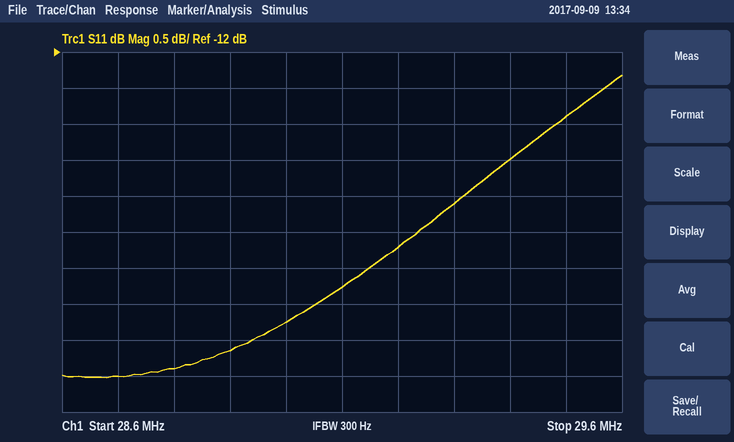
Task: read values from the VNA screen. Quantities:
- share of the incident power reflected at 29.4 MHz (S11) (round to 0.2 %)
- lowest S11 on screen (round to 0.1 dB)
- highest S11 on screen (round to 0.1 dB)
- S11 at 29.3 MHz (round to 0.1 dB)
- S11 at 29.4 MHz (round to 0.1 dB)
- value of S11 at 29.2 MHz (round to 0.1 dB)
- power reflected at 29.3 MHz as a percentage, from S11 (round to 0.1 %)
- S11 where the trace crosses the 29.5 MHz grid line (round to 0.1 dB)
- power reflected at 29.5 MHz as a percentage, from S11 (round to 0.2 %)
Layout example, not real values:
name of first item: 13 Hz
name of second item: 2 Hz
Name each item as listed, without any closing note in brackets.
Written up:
share of the incident power reflected at 29.4 MHz (S11): 4.4 %
lowest S11 on screen: -16.5 dB
highest S11 on screen: -12.3 dB
S11 at 29.3 MHz: -14.1 dB
S11 at 29.4 MHz: -13.5 dB
value of S11 at 29.2 MHz: -14.7 dB
power reflected at 29.3 MHz as a percentage, from S11: 3.9 %
S11 where the trace crosses the 29.5 MHz grid line: -12.9 dB
power reflected at 29.5 MHz as a percentage, from S11: 5.2 %
